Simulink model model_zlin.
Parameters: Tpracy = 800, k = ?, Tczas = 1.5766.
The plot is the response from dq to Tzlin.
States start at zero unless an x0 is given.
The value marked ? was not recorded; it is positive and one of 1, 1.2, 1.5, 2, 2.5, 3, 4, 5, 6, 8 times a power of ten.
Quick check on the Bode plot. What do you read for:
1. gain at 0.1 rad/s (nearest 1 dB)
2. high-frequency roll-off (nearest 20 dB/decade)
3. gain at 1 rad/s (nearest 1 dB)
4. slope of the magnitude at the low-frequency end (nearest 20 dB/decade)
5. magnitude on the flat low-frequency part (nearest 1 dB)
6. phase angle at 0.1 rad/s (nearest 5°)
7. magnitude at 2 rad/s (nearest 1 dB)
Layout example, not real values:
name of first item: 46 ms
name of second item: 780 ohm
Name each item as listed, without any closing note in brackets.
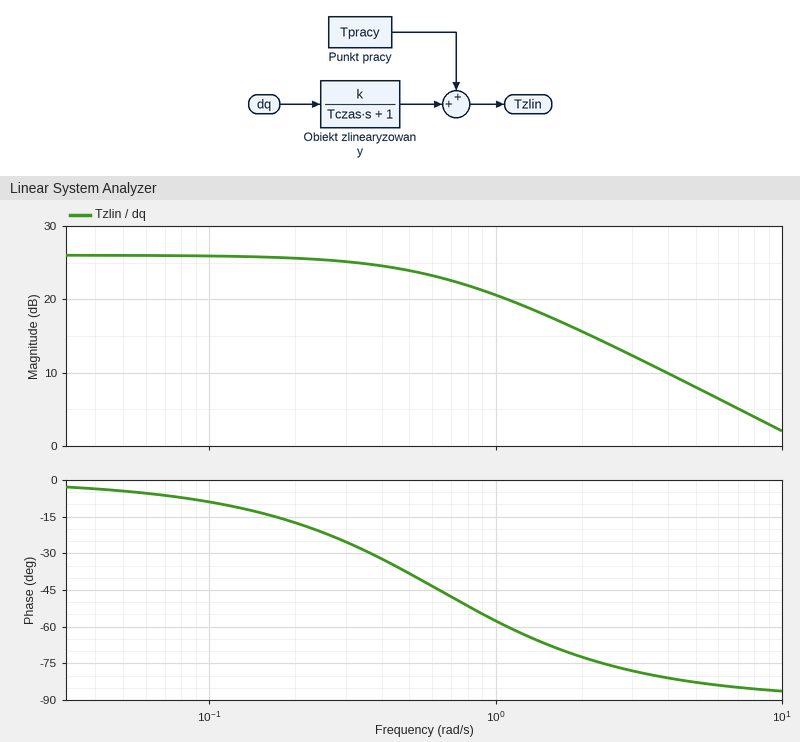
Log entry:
gain at 0.1 rad/s: 26 dB
high-frequency roll-off: -20 dB/decade
gain at 1 rad/s: 21 dB
slope of the magnitude at the low-frequency end: 0 dB/decade
magnitude on the flat low-frequency part: 26 dB
phase angle at 0.1 rad/s: -10°
magnitude at 2 rad/s: 16 dB
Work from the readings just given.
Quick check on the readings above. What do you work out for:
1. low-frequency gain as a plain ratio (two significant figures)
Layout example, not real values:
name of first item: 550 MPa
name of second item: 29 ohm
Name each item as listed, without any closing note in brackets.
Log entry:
low-frequency gain as a plain ratio: 20
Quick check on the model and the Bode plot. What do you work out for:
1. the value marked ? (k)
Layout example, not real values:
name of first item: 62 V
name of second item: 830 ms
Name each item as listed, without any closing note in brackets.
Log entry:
the value marked ?: 20
